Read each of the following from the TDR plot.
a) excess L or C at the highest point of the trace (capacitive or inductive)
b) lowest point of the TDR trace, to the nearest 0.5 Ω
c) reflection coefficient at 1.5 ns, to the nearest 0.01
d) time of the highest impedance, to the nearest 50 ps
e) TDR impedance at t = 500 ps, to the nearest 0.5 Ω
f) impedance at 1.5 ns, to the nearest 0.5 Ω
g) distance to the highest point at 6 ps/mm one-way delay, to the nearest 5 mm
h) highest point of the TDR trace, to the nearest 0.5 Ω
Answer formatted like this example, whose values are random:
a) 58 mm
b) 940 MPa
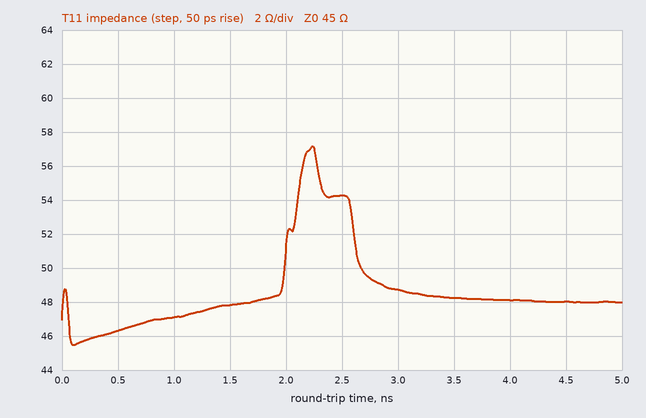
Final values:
a) inductive
b) 45.5 Ω
c) +0.03
d) 2.25 ns
e) 46.5 Ω
f) 48.0 Ω
g) 185 mm
h) 57.0 Ω
